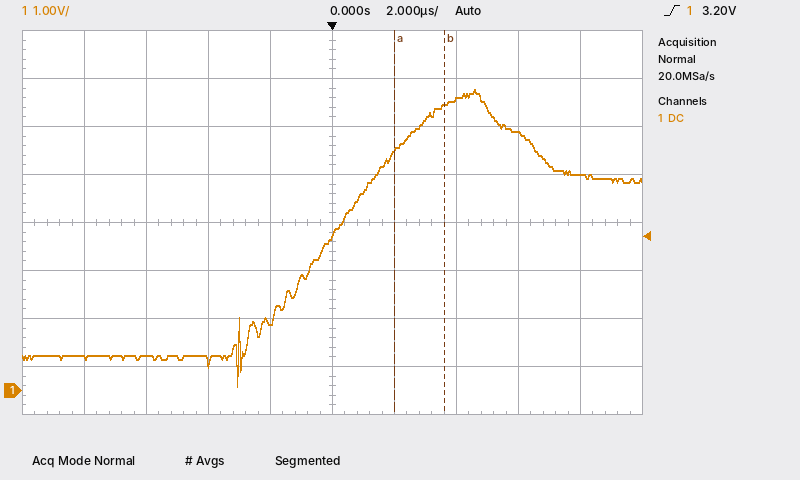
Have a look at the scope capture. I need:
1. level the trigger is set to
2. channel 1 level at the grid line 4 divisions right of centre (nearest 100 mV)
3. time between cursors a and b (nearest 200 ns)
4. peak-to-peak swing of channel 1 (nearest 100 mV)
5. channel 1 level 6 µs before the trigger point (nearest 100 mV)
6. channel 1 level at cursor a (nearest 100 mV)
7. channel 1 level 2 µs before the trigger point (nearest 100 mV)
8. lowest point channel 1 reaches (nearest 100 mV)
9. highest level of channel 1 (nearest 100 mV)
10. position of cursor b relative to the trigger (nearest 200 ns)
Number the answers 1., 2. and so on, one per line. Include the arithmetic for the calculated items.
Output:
1. 3.20 V
2. 4.5 V
3. 1.6 µs
4. 6.3 V − (100 mV) = 6.2 V
5. 700 mV
6. 5.0 V
7. 1.4 V
8. 100 mV
9. 6.3 V
10. +3.6 µs
